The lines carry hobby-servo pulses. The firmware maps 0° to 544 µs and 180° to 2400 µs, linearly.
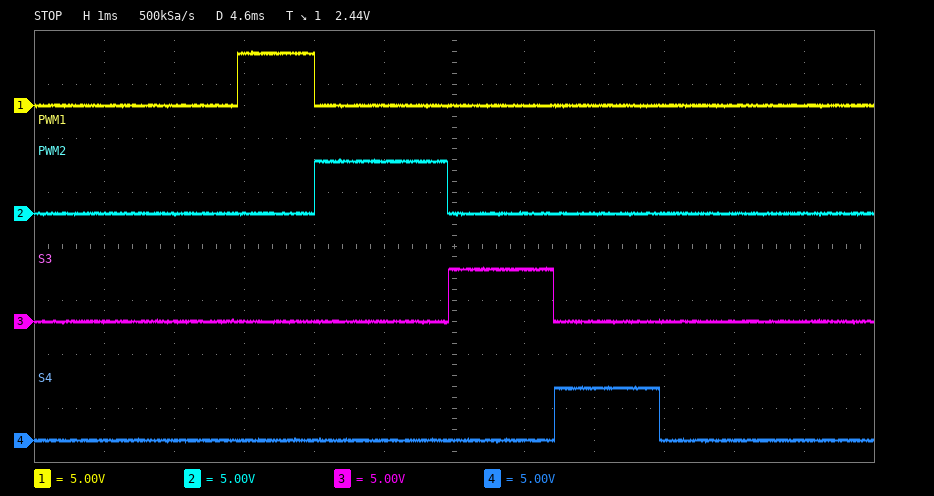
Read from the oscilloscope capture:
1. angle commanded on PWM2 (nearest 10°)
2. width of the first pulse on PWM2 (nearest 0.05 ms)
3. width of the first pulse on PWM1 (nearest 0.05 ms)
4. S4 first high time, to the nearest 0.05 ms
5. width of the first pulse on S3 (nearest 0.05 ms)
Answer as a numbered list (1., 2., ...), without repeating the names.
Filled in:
1. 130°
2. 1.90 ms
3. 1.10 ms
4. 1.50 ms
5. 1.50 ms
